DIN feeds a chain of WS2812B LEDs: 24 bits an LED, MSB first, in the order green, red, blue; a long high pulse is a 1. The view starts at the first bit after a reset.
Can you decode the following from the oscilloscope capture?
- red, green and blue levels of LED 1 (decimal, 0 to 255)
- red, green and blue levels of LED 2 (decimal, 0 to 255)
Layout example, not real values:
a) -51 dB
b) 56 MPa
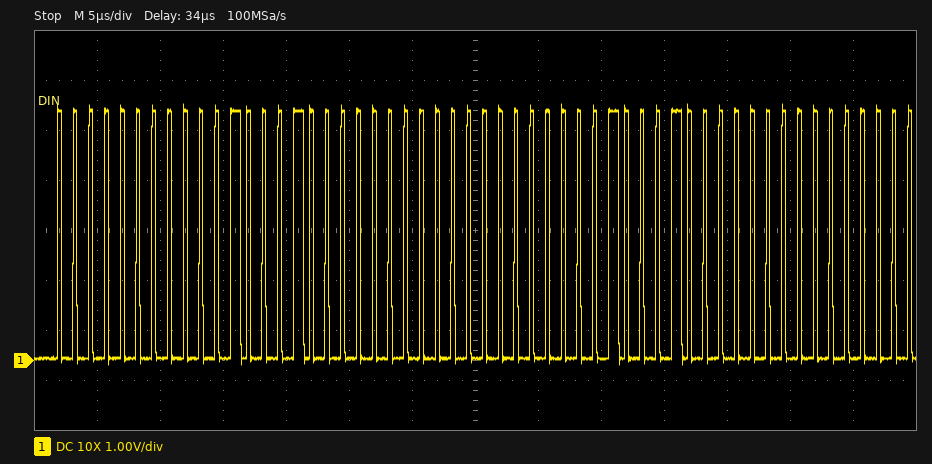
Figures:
a) 17, 0, 0
b) 17, 0, 0
